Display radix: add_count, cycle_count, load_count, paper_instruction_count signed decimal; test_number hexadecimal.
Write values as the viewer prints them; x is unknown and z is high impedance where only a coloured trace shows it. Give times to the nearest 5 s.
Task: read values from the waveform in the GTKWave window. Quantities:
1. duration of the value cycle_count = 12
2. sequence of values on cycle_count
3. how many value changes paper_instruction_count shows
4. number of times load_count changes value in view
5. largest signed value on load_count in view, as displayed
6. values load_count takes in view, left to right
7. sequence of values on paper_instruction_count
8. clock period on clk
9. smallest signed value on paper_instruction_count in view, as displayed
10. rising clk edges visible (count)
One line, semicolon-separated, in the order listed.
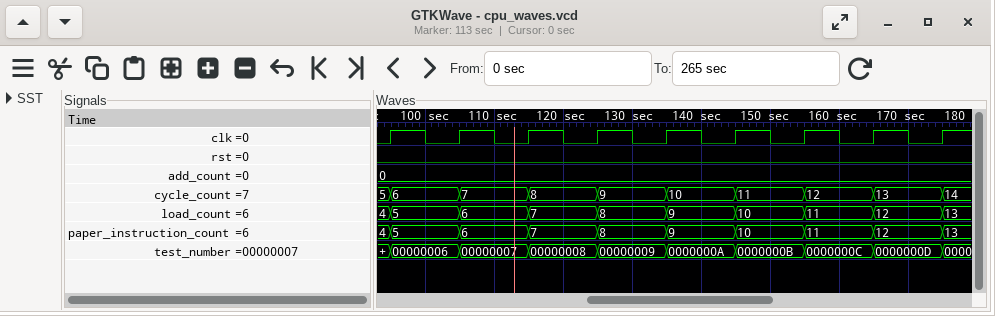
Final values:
10 s; 5, 6, 7, 8, 9, 10, 11, 12, 13, 14; 9; 9; 13; 4, 5, 6, 7, 8, 9, 10, 11, 12, 13; 4, 5, 6, 7, 8, 9, 10, 11, 12, 13; 10 s; 4; 9
